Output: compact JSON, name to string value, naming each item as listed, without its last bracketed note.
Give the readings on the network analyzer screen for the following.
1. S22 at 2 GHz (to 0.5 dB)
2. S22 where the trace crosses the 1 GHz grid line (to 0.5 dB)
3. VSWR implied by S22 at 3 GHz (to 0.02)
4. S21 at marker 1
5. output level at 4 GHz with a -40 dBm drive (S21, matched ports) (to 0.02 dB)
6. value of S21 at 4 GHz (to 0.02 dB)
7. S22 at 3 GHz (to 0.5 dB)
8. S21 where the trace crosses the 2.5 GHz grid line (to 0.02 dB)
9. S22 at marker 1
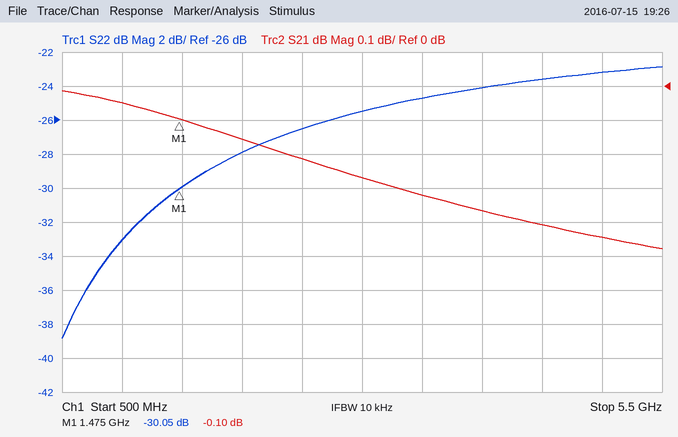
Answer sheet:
{"S22 at 2 GHz": "-28.0 dB", "S22 where the trace crosses the 1 GHz grid line": "-33.0 dB", "VSWR implied by S22 at 3 GHz": "1.12", "S21 at marker 1": "-0.10 dB", "output level at 4 GHz with a -40 dBm drive (S21, matched ports)": "-40.36 dBm", "value of S21 at 4 GHz": "-0.36 dB", "S22 at 3 GHz": "-25.5 dB", "S21 where the trace crosses the 2.5 GHz grid line": "-0.22 dB", "S22 at marker 1": "-30.05 dB"}
